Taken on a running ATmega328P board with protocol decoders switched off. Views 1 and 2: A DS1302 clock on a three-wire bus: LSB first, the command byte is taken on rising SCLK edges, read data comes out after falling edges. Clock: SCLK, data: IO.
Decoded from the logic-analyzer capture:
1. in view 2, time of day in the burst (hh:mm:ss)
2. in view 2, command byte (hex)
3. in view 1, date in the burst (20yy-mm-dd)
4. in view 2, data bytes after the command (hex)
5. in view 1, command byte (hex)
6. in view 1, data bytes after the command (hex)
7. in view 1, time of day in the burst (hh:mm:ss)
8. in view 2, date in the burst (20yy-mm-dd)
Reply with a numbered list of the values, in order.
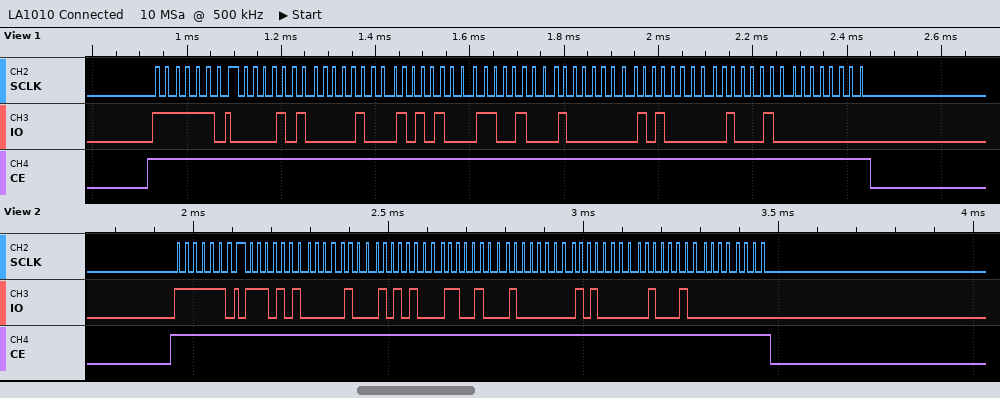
1. 15:10:57
2. 0xBF
3. 2022-01-13
4. 57 10 15 13 01 05 22 00
5. 0xBF
6. 50 10 15 13 01 05 22 00
7. 15:10:50
8. 2022-01-13
